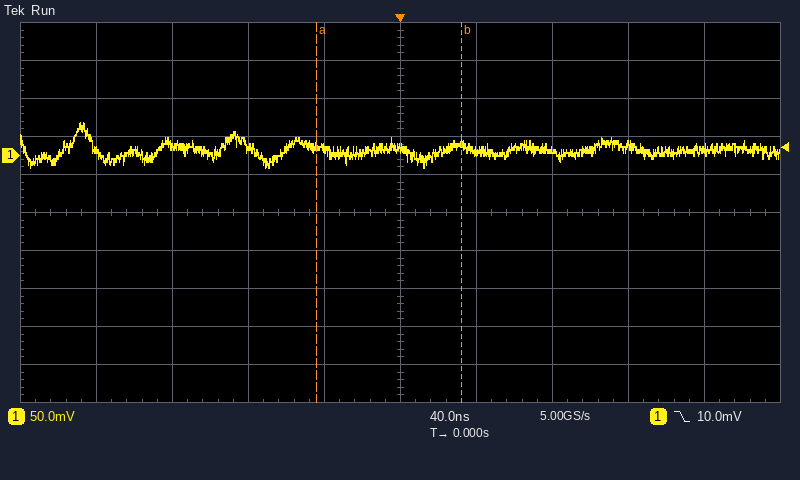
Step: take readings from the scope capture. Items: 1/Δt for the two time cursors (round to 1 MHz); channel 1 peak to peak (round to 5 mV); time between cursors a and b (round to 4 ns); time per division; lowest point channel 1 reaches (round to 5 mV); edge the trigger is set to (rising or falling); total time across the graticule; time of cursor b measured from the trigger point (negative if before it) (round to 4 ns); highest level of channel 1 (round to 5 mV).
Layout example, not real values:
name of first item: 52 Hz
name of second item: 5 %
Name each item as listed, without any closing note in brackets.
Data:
1/Δt for the two time cursors: 13 MHz
channel 1 peak to peak: 60 mV
time between cursors a and b: 76 ns
time per division: 40 ns
lowest point channel 1 reaches: -15 mV
edge the trigger is set to: falling
total time across the graticule: 400 ns
time of cursor b measured from the trigger point (negative if before it): +32 ns
highest level of channel 1: 45 mV
